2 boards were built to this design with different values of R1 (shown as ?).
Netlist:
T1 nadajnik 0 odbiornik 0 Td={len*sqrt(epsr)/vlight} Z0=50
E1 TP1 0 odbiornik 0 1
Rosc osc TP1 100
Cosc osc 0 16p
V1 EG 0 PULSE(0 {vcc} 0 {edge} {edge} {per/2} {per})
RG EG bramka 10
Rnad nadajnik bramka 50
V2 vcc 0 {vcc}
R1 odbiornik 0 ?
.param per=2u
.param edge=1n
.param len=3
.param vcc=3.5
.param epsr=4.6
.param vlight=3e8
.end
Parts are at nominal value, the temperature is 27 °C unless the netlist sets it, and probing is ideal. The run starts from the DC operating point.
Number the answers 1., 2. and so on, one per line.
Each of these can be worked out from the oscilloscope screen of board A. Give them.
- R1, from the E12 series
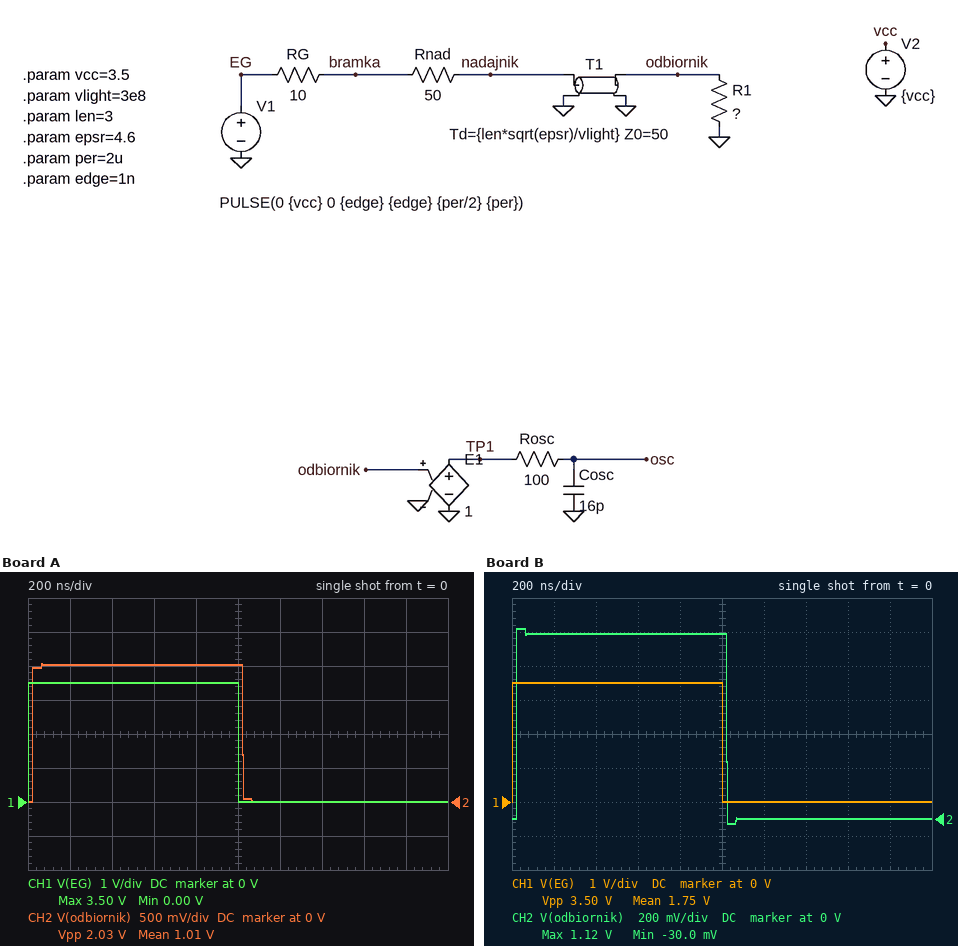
1. 82 Ω
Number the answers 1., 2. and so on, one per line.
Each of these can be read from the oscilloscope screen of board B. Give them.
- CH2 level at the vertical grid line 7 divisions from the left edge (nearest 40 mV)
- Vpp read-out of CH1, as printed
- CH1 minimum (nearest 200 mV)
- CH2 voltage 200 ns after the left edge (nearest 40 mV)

1. 0 V
2. 3.50 V
3. 0 V
4. 1.08 V
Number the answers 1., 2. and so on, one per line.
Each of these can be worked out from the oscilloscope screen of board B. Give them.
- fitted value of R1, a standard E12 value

1. 27 Ω
